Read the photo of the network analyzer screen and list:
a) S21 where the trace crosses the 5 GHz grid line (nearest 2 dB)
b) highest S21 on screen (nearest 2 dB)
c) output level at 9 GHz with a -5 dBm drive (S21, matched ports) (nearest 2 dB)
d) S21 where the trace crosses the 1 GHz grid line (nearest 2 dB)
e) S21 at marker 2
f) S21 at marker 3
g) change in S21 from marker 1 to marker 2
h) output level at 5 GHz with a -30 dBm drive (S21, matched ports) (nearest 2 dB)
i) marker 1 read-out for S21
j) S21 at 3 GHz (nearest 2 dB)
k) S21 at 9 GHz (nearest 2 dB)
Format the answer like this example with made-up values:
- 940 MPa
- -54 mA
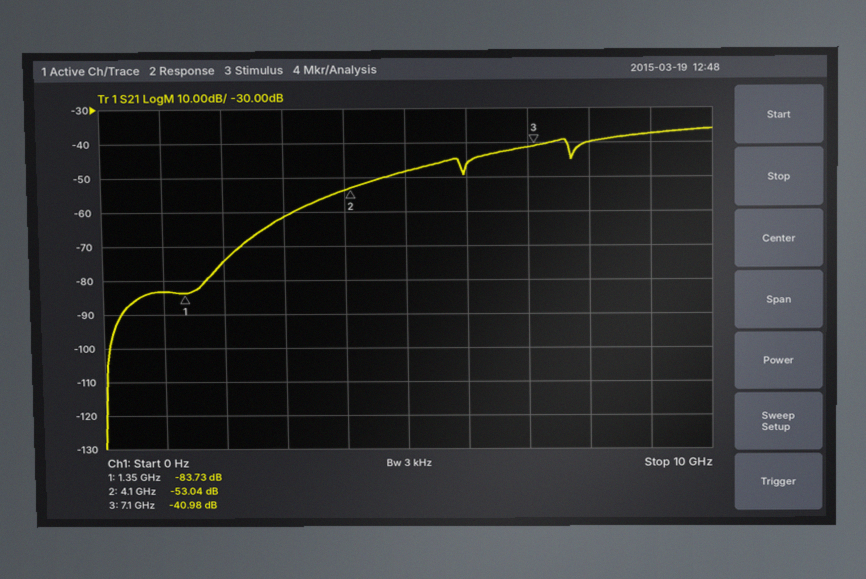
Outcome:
- -48 dB
- -36 dB
- -42 dBm
- -84 dB
- -53.04 dB
- -40.98 dB
- 30.69 dB
- -78 dBm
- -83.73 dB
- -62 dB
- -38 dB
